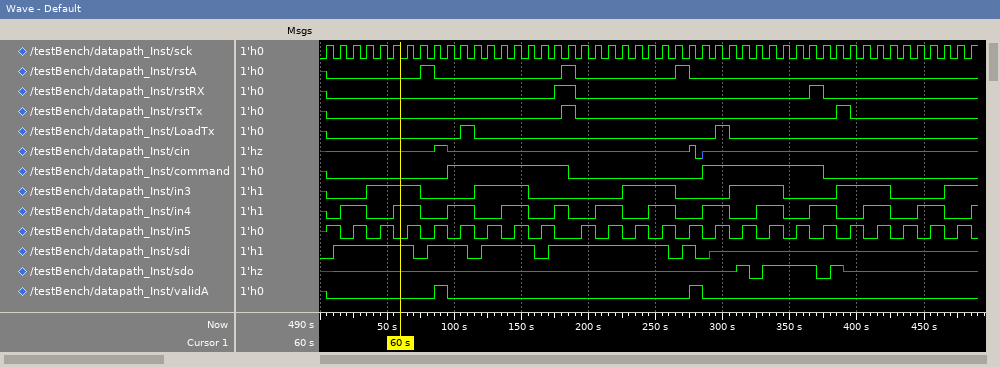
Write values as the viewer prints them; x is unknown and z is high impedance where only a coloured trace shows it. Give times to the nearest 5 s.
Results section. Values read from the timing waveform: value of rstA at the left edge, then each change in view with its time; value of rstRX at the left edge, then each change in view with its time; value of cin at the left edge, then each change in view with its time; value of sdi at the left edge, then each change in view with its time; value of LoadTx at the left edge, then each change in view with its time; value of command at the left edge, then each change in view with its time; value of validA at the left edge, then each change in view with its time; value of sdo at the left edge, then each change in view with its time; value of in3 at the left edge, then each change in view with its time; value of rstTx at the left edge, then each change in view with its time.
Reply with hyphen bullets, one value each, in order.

- x, 0 at 5 s, 1 at 75 s, 0 at 85 s, 1 at 180 s, 0 at 190 s, 1 at 265 s, 0 at 275 s
- x, 0 at 5 s, 1 at 175 s, 0 at 190 s, 1 at 365 s, 0 at 375 s
- x, z at 5 s, 1 at 85 s, z at 95 s, 1 at 275 s, 0 at 280 s, z at 285 s
- 0, 1 at 10 s, 0 at 70 s, 1 at 80 s, 0 at 110 s, 1 at 120 s, 0 at 160 s, 1 at 170 s, 0 at 260 s, 1 at 270 s, 0 at 280 s, z at 290 s
- x, 0 at 5 s, 1 at 105 s, 0 at 115 s, 1 at 295 s, 0 at 305 s
- x, 0 at 5 s, 1 at 95 s, 0 at 185 s, 1 at 285 s, 0 at 375 s
- x, 0 at 5 s, 1 at 85 s, 0 at 95 s, 1 at 275 s, 0 at 285 s
- x, z at 10 s, 1 at 310 s, 0 at 320 s, 1 at 330 s, 0 at 370 s, 1 at 380 s, z at 390 s
- x, 0 at 5 s, 1 at 35 s, 0 at 75 s, 1 at 115 s, 0 at 155 s, 1 at 225 s, 0 at 265 s, 1 at 305 s, 0 at 345 s, 1 at 385 s, 0 at 425 s, 1 at 465 s
- x, 0 at 5 s, 1 at 180 s, 0 at 190 s, 1 at 385 s, 0 at 395 s
